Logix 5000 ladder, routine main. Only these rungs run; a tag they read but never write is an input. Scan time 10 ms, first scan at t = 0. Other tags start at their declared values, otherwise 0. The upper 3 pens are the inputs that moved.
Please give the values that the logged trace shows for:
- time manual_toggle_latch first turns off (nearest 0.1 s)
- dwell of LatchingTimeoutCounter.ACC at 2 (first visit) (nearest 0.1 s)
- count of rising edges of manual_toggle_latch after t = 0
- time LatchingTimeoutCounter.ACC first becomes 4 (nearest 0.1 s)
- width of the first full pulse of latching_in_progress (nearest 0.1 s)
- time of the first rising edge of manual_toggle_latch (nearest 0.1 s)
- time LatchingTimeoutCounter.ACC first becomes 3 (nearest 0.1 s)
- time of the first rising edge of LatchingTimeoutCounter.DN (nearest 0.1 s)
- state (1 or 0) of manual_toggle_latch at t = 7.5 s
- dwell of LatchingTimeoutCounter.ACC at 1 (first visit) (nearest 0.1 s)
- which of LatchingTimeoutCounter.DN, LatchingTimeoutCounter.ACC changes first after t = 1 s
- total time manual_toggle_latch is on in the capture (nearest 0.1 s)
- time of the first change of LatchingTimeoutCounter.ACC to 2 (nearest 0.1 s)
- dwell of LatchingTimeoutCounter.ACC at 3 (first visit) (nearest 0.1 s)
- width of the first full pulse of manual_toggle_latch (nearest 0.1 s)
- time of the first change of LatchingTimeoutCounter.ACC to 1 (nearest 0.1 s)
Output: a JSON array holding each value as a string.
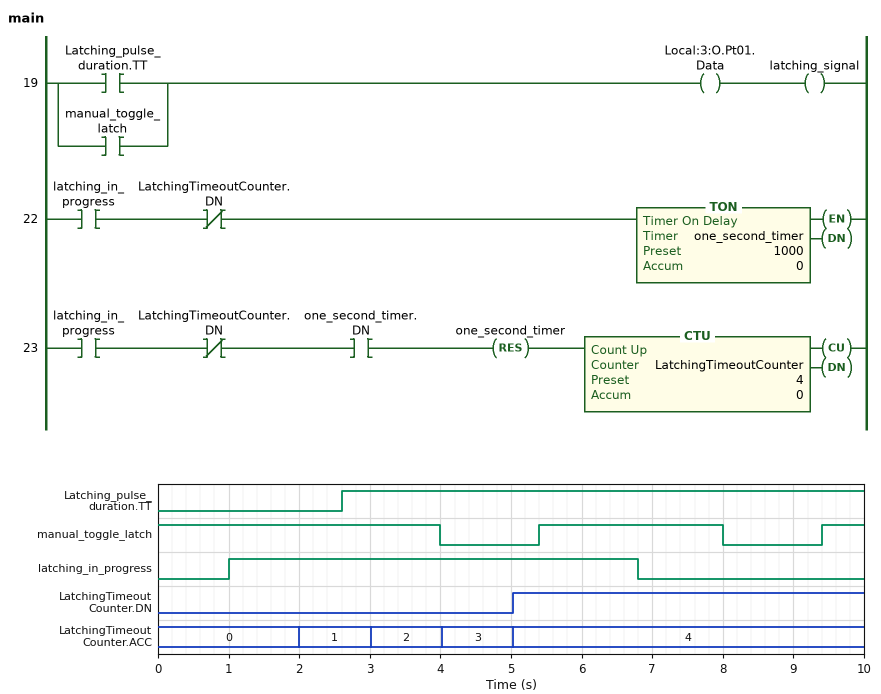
["4.0 s", "1.0 s", "2", "5.0 s", "5.8 s", "5.4 s", "4.0 s", "5.0 s", "1", "1.0 s", "LatchingTimeoutCounter.ACC", "7.2 s", "3.0 s", "1.0 s", "2.6 s", "2.0 s"]
